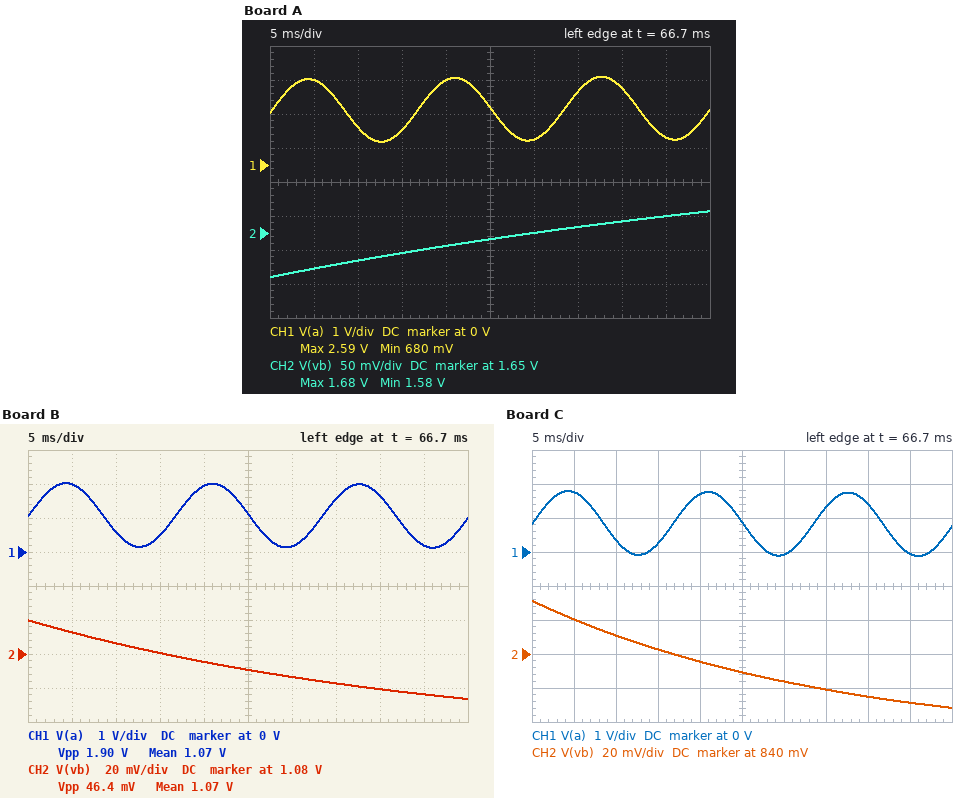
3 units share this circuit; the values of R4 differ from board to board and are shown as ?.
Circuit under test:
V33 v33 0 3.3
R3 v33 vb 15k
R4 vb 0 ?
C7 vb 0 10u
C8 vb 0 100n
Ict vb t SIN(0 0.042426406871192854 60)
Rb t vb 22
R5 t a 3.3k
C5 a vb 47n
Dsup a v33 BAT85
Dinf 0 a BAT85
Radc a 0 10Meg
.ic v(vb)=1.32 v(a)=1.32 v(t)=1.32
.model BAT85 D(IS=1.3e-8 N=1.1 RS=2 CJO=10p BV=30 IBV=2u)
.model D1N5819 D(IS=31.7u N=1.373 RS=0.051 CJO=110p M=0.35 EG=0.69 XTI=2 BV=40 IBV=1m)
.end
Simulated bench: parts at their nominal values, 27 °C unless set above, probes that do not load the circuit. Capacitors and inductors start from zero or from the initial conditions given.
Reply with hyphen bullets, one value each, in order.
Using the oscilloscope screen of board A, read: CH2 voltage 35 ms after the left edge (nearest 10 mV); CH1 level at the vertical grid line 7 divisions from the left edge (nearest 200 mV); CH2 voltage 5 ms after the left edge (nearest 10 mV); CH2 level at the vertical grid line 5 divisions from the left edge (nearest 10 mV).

- 1.66 V
- 2.2 V
- 1.60 V
- 1.64 V
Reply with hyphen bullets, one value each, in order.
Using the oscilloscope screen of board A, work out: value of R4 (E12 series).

- 18 kΩ
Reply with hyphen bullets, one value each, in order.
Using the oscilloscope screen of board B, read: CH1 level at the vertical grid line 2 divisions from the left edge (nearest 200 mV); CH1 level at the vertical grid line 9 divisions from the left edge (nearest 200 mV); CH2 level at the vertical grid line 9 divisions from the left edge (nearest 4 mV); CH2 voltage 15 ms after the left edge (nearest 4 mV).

- 600 mV
- 200 mV
- 1.056 V
- 1.080 V
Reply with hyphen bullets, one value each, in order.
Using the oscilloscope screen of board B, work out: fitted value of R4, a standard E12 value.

- 6.8 kΩ
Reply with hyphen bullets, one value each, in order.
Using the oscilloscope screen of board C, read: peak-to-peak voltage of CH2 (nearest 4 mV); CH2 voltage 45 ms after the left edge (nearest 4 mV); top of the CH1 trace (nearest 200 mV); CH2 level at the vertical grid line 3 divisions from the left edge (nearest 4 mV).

- 64 mV
- 812 mV
- 1.8 V
- 844 mV
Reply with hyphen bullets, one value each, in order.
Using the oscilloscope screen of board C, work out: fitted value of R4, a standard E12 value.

- 4.7 kΩ
